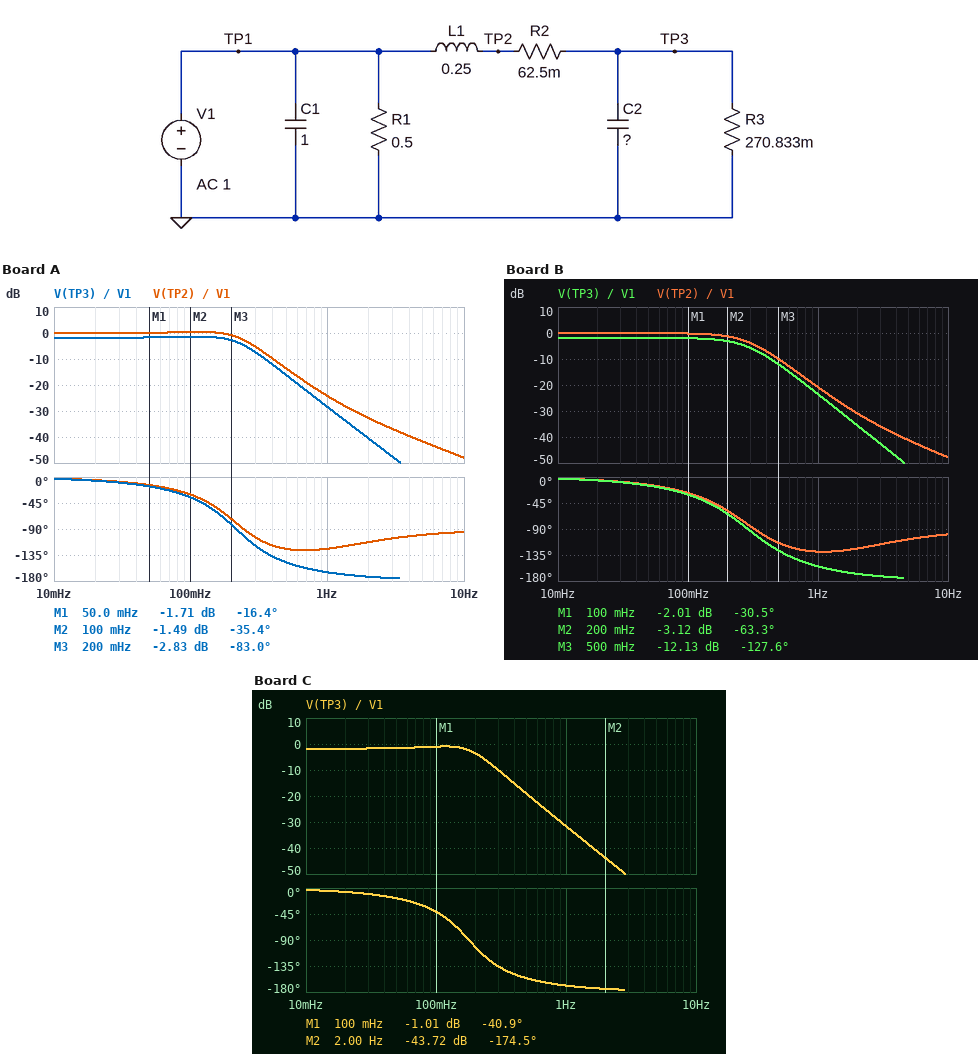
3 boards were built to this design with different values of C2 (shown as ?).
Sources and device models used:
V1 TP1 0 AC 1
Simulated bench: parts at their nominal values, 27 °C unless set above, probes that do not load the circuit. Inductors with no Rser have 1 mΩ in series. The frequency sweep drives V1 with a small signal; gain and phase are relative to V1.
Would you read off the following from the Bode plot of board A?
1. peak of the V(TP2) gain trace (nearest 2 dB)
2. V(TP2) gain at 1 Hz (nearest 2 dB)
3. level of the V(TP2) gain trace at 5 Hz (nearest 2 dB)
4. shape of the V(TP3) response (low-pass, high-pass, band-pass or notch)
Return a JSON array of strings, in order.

["0 dB", "-24 dB", "-42 dB", "low-pass"]
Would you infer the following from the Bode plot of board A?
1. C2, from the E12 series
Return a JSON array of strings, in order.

["2.7 F"]
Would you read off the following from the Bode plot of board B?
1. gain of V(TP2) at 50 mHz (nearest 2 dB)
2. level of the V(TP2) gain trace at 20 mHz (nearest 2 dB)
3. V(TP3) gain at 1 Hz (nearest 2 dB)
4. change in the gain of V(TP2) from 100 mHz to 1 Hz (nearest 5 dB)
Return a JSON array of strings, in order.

["0 dB", "0 dB", "-24 dB", "-20 dB"]
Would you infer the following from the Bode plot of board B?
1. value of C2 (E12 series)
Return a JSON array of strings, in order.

["1.5 F"]
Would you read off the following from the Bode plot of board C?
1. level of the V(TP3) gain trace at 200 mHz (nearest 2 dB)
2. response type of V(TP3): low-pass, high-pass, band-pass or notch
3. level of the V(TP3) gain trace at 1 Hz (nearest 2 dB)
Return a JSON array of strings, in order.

["-4 dB", "low-pass", "-32 dB"]
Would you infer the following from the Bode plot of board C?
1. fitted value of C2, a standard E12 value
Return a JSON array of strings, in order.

["3.9 F"]
